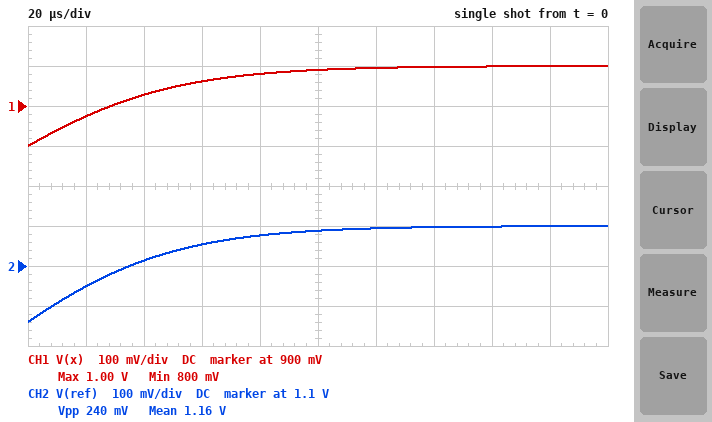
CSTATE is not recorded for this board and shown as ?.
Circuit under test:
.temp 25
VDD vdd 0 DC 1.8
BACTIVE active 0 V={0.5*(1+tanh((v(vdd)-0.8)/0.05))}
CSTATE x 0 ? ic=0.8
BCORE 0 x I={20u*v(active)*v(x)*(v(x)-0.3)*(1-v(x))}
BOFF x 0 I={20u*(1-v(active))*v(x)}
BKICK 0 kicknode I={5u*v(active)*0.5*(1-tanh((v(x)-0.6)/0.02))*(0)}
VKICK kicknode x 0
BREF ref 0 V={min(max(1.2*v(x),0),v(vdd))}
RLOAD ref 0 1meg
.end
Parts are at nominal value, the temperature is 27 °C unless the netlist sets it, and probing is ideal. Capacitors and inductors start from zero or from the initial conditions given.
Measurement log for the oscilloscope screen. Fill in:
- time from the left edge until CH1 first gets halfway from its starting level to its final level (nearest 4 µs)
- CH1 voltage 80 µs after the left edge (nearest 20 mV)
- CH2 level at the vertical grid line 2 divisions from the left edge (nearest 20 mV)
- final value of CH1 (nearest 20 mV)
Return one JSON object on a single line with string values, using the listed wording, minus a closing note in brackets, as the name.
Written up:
{"time from the left edge until CH1 first gets halfway from its starting level to its final level": "28 µs", "CH1 voltage 80 µs after the left edge": "980 mV", "CH2 level at the vertical grid line 2 divisions from the left edge": "1.12 V", "final value of CH1": "1.00 V"}
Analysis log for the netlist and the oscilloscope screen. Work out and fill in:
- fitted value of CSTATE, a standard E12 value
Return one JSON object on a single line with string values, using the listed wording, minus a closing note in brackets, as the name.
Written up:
{"fitted value of CSTATE, a standard E12 value": "390 pF"}
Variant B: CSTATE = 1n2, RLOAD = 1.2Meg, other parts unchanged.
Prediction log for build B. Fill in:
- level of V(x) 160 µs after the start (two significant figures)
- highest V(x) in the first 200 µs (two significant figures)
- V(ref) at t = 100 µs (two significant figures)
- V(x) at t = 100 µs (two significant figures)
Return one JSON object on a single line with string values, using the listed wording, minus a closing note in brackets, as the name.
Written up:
{"level of V(x) 160 µs after the start": "950 mV", "highest V(x) in the first 200 µs": "970 mV", "V(ref) at t = 100 µs": "1.1 V", "V(x) at t = 100 µs": "910 mV"}
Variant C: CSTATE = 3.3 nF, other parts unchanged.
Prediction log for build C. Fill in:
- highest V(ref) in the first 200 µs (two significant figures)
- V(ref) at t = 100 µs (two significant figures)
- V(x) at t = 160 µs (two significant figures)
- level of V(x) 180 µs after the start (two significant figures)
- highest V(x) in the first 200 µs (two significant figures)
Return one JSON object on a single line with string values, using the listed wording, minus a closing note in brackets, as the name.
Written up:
{"highest V(ref) in the first 200 µs": "1.1 V", "V(ref) at t = 100 µs": "1.0 V", "V(x) at t = 160 µs": "870 mV", "level of V(x) 180 µs after the start": "880 mV", "highest V(x) in the first 200 µs": "890 mV"}
